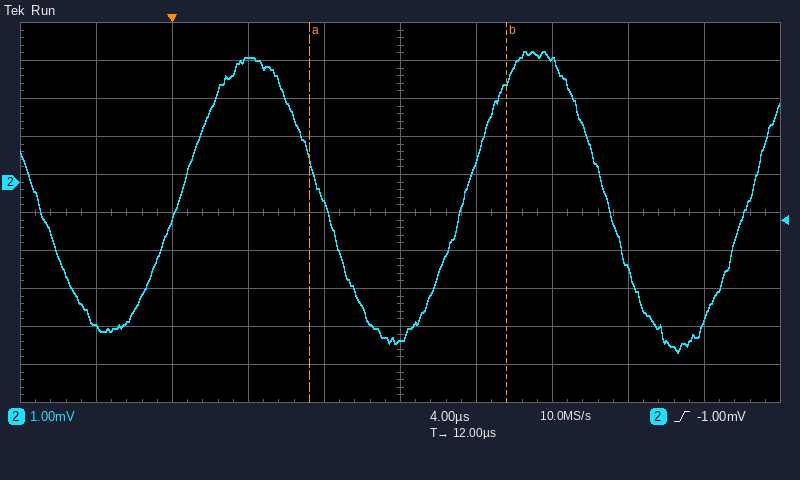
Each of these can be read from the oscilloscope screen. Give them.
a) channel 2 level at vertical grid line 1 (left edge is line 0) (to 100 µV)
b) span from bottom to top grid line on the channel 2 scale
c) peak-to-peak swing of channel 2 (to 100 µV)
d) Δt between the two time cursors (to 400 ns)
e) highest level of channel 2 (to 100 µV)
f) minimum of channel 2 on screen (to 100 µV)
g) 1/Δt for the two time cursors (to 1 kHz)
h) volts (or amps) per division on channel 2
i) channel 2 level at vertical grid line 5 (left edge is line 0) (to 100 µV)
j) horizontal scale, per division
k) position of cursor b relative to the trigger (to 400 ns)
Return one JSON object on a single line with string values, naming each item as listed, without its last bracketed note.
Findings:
{"channel 2 level at vertical grid line 1 (left edge is line 0)": "-3.8 mV", "span from bottom to top grid line on the channel 2 scale": "10 mV", "peak-to-peak swing of channel 2": "7.9 mV", "Δt between the two time cursors": "10.4 µs", "highest level of channel 2": "3.4 mV", "minimum of channel 2 on screen": "-4.5 mV", "1/Δt for the two time cursors": "96 kHz", "volts (or amps) per division on channel 2": "1 mV", "channel 2 level at vertical grid line 5 (left edge is line 0)": "-4.2 mV", "horizontal scale, per division": "4 µs", "position of cursor b relative to the trigger": "+17.6 µs"}
